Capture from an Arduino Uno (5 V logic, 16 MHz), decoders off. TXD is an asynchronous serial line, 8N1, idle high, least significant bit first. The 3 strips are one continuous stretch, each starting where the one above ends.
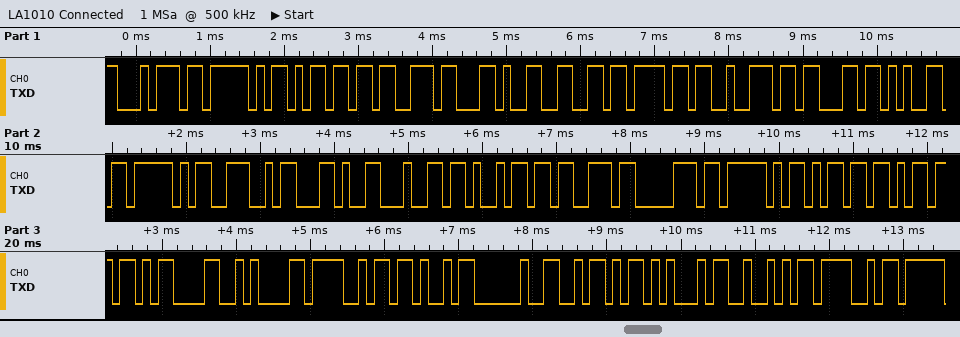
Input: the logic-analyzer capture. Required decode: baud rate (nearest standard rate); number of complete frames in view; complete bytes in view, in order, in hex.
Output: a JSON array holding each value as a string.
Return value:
["9600 baud", "29", "0x74 0x5F 0x6D 0x73 0x2C 0x66 0x6F 0x72 0x63 0x65 0x5F 0x4E 0x2C 0x64 0x69 0x73 0x70 0x5F 0x6D 0x6D 0x0D 0x0A 0x4F 0x4B 0x20 0x5A 0x45 0x52 0x4F"]
